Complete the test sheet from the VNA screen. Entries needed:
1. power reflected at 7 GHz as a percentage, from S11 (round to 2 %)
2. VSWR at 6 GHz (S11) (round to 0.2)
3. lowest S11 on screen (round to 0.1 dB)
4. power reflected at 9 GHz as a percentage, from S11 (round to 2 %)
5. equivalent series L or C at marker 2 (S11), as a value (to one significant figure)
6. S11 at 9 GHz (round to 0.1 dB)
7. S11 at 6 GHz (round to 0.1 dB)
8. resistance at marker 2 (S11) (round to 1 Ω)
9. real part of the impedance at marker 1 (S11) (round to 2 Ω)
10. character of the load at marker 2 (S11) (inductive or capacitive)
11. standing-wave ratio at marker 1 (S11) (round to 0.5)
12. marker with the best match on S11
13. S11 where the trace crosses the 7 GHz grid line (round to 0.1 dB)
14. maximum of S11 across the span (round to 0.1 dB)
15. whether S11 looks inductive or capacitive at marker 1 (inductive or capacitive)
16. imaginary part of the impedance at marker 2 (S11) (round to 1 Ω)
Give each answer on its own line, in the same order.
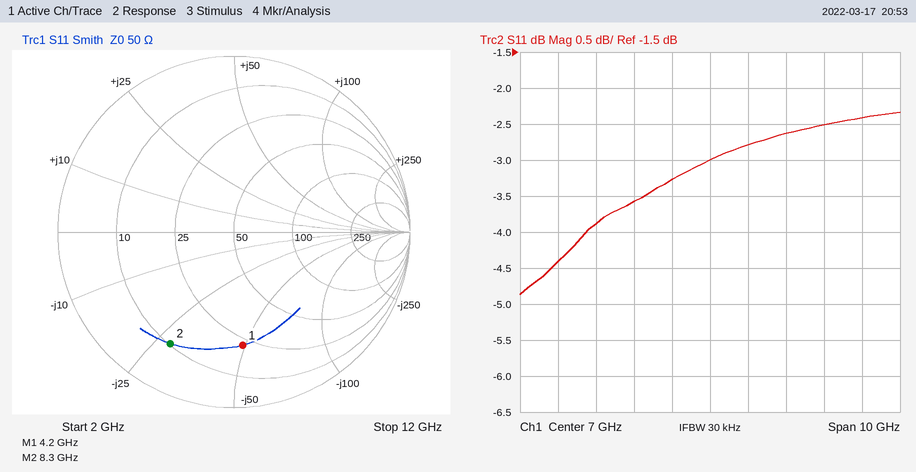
50 %
5.4
-4.9 dB
54 %
700 fF
-2.6 dB
-3.3 dB
10 Ω
22 Ω
capacitive
4.5
marker 1
-3.0 dB
-2.3 dB
capacitive
-28 Ω
